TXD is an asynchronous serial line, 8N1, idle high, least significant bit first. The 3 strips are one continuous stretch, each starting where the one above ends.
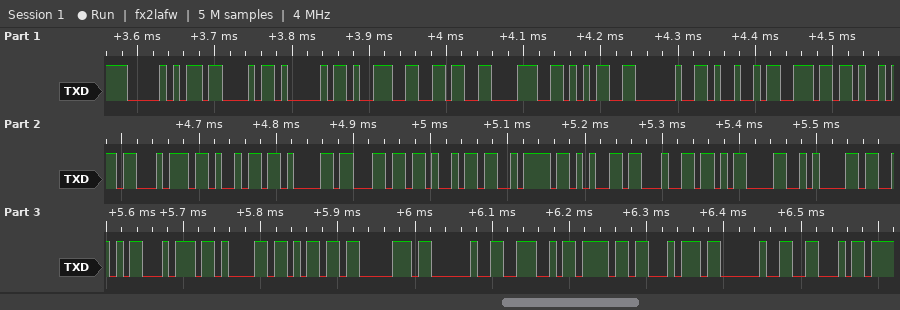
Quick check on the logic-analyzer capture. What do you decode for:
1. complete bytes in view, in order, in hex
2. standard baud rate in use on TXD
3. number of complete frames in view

50 43 41 39 36 38 35 20 49 6E 69 74 69 61 6C 69 7A 65 64 0D 0A 53 74 61 6D 70 20 4E 6F 74 20 46
115200 baud
32
